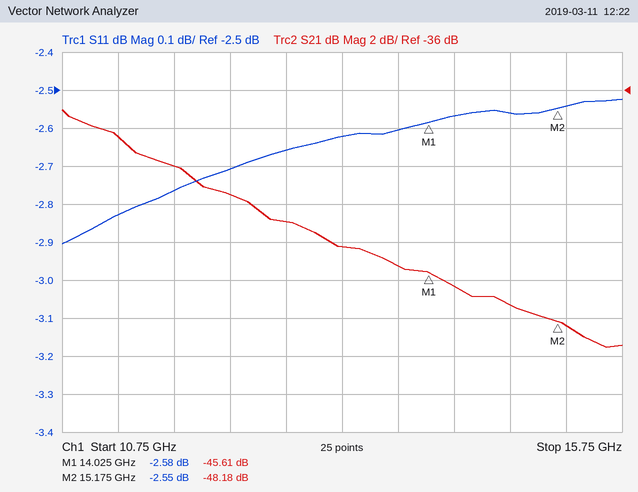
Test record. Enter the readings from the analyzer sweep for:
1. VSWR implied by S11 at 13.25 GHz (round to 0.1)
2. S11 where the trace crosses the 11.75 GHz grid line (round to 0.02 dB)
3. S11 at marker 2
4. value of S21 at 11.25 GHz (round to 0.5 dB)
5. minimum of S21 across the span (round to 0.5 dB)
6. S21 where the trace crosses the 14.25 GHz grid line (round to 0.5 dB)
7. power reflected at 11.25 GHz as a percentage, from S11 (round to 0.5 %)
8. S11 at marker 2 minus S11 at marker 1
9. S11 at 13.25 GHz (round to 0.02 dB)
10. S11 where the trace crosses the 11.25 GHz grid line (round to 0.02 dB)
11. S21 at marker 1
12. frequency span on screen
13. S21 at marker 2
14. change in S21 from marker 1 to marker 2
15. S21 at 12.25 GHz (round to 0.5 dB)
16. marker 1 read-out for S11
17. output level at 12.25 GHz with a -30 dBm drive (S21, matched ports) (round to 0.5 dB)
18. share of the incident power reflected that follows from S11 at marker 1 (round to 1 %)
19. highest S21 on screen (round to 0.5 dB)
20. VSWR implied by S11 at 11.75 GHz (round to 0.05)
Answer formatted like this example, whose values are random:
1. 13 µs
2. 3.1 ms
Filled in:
1. 6.7
2. -2.76 dB
3. -2.55 dB
4. -38.5 dB
5. -49.5 dB
6. -46.5 dB
7. 52.0 %
8. 0.03 dB
9. -2.62 dB
10. -2.82 dB
11. -45.61 dB
12. 5 GHz
13. -48.18 dB
14. -2.57 dB
15. -41.5 dB
16. -2.58 dB
17. -71.5 dBm
18. 55 %
19. -37.0 dB
20. 6.35
